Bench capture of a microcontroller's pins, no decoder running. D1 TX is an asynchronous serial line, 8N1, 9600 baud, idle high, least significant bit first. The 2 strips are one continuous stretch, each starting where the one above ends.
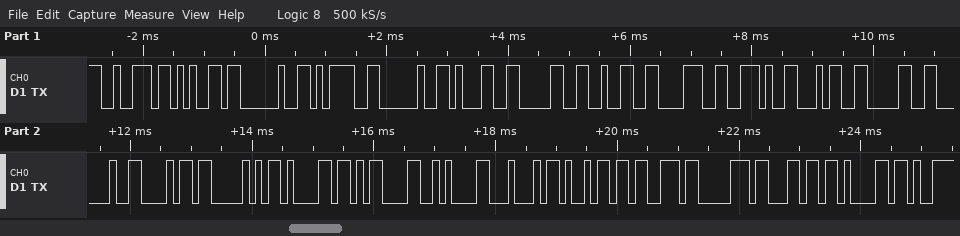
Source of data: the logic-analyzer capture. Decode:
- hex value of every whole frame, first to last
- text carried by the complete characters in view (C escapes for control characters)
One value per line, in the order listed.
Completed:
72 65 20 3D 20 31 30 32 38 2E 34 30 20 68 50 61 0D 0A 44 69 73 70 6C 61
"re = 1028.40 hPa\r\nDispla"
